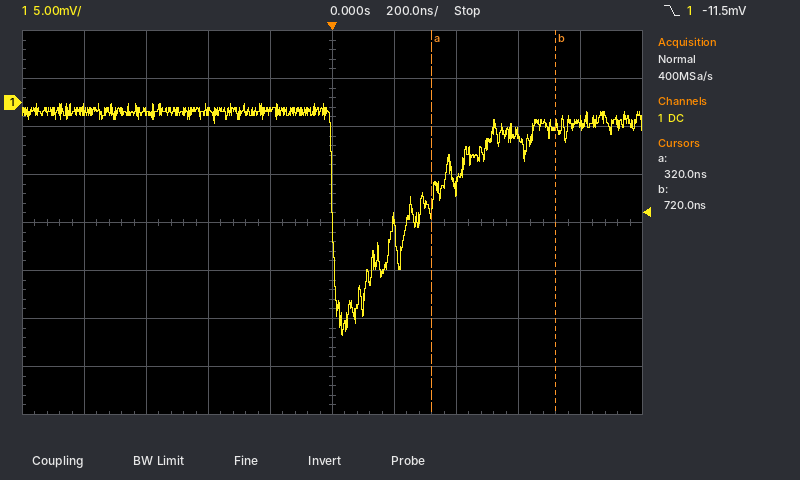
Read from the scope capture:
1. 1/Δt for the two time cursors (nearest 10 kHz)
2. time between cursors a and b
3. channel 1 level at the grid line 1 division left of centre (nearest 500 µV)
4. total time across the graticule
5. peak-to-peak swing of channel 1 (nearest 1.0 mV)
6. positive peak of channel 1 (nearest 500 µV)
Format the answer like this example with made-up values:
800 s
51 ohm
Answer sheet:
2.50 MHz
400 ns
-1.0 mV
2 µs
24.0 mV
0.0 mV
